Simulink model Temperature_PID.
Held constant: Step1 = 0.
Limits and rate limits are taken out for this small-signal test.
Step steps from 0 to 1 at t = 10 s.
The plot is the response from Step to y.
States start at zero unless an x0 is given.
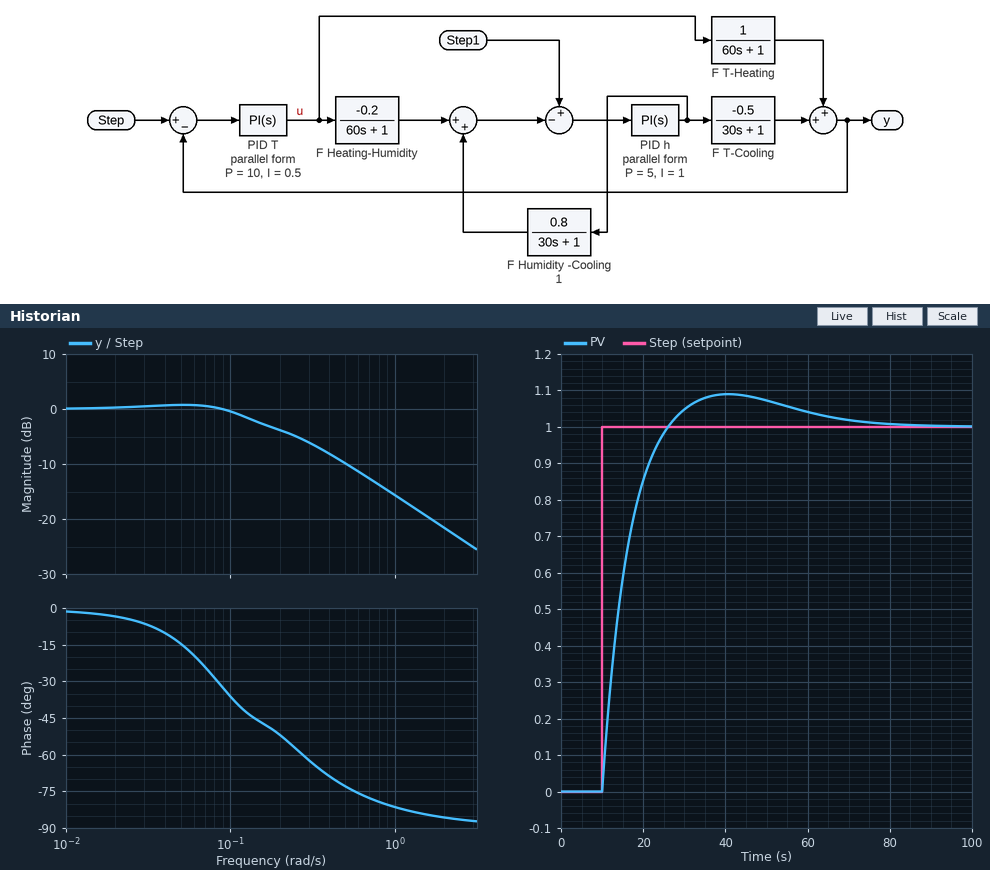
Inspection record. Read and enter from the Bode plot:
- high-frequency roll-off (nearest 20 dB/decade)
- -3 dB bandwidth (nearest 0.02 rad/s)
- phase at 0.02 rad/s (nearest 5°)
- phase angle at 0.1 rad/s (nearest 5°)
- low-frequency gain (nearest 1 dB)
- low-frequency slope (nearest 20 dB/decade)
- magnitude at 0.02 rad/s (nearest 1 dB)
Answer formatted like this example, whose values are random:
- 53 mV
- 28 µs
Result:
- -20 dB/decade
- 0.16 rad/s
- -5°
- -35°
- 0 dB
- 0 dB/decade
- 0 dB
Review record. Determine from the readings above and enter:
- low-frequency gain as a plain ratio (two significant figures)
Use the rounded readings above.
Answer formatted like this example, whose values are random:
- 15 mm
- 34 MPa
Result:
- 1.0
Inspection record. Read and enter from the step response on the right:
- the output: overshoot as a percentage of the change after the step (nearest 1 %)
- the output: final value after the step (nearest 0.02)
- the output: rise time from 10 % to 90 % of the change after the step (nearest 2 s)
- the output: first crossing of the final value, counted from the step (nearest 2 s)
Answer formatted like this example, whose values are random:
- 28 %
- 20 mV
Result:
- 9 %
- 1.00
- 10 s
- 16 s
